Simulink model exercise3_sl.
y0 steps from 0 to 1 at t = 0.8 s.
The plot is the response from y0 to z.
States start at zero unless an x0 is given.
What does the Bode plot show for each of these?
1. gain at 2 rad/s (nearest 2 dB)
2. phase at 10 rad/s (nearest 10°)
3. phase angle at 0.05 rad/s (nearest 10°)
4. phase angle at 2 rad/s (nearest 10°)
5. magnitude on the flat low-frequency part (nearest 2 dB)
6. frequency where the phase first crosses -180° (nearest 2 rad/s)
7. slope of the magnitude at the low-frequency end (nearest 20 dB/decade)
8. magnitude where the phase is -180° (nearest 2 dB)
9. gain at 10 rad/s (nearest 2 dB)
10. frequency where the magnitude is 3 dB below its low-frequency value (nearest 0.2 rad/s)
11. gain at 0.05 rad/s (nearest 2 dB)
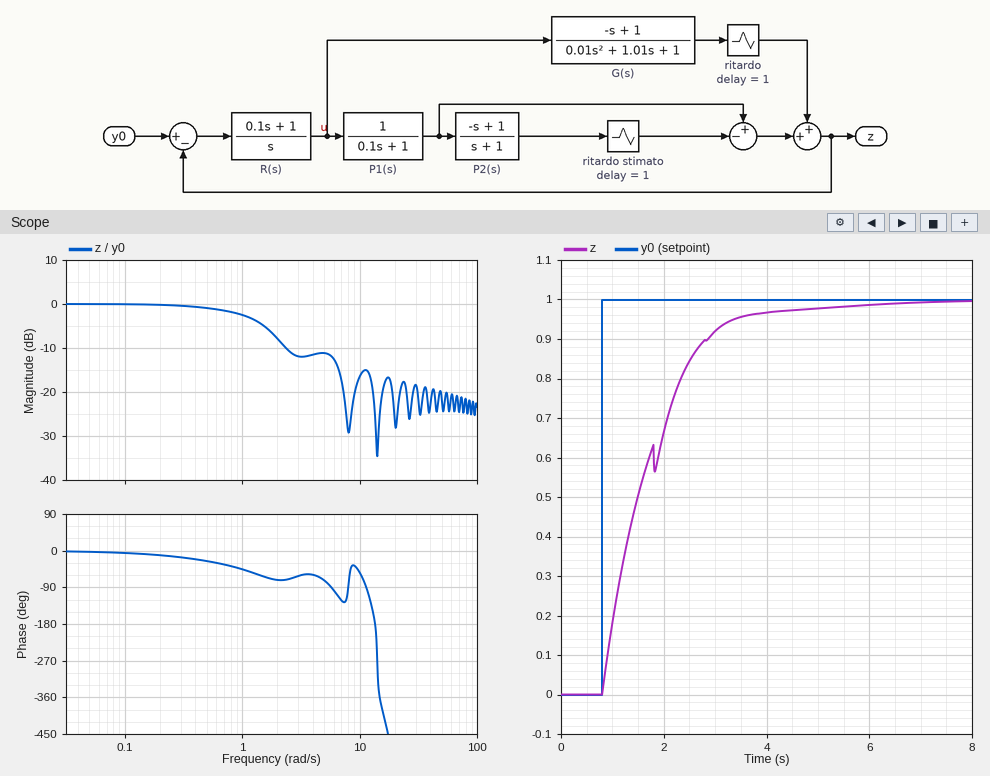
-8 dB
-50°
0°
-70°
0 dB
14 rad/s
0 dB/decade
-26 dB
-16 dB
1.2 rad/s
0 dB
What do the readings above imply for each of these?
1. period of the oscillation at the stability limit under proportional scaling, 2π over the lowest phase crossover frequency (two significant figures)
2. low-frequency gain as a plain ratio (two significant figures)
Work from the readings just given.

0.45 s
1.0
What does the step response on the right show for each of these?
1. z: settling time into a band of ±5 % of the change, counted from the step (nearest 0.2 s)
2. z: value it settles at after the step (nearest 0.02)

2.6 s
1.00
